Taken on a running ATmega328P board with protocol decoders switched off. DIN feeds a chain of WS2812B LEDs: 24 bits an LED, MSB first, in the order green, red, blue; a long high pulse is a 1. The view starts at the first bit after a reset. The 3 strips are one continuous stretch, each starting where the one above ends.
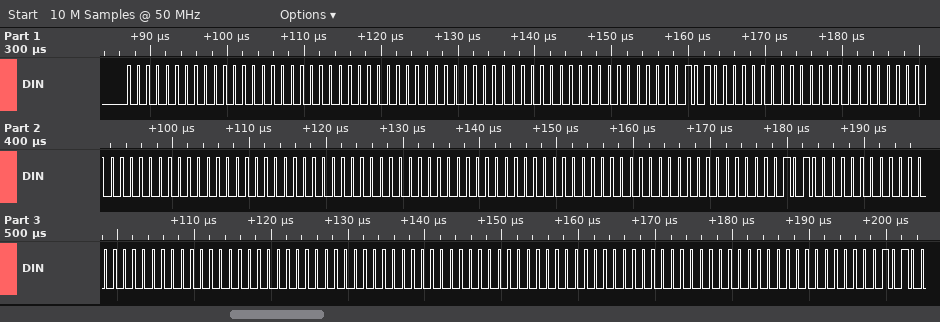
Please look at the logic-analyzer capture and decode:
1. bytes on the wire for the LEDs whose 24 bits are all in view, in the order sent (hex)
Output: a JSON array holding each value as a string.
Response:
["00 00 00 00 00 00 00 28 00 00 00 00 00 00 00 00 00 00 00 28 00 00 00 00 00 00 00 00 00 00"]
